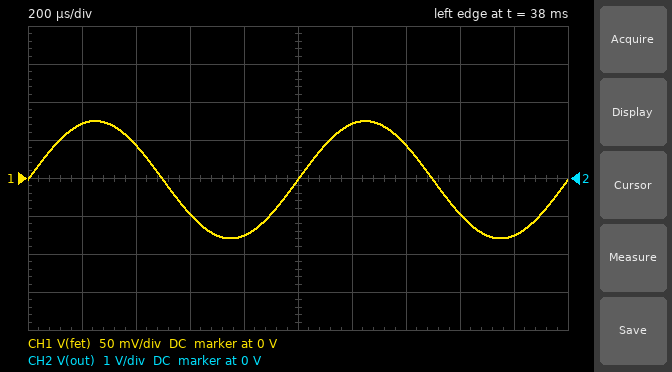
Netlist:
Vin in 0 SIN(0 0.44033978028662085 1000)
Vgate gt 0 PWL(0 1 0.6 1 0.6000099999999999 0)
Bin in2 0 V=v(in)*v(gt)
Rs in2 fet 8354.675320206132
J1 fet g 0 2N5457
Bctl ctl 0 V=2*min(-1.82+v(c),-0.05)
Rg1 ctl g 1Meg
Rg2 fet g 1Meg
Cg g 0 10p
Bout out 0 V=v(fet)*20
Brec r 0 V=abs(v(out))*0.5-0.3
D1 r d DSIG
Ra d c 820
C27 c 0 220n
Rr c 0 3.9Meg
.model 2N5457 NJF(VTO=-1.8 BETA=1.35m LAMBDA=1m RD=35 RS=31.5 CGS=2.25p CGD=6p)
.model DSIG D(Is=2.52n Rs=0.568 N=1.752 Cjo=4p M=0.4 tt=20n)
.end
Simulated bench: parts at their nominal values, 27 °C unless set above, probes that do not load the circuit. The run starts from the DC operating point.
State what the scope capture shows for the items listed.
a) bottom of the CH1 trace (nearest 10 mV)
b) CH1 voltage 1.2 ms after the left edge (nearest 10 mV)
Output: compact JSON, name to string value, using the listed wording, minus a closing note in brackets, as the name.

{"bottom of the CH1 trace": "-80 mV", "CH1 voltage 1.2 ms after the left edge": "70 mV"}
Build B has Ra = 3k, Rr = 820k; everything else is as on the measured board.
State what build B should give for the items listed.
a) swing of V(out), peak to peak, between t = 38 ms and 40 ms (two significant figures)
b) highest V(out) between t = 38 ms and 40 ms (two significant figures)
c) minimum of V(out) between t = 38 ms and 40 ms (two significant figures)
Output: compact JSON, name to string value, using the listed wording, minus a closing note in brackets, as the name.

{"swing of V(out), peak to peak, between t = 38 ms and 40 ms": "3.2 V", "highest V(out) between t = 38 ms and 40 ms": "1.6 V", "minimum of V(out) between t = 38 ms and 40 ms": "-1.7 V"}
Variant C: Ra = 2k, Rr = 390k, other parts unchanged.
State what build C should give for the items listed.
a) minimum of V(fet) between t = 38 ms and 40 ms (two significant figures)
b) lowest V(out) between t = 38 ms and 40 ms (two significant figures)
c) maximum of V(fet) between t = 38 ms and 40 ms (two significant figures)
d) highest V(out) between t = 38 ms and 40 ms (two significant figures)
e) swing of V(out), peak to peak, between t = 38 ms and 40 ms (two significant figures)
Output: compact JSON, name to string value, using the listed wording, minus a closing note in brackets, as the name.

{"minimum of V(fet) between t = 38 ms and 40 ms": "-86 mV", "lowest V(out) between t = 38 ms and 40 ms": "-1.7 V", "maximum of V(fet) between t = 38 ms and 40 ms": "81 mV", "highest V(out) between t = 38 ms and 40 ms": "1.6 V", "swing of V(out), peak to peak, between t = 38 ms and 40 ms": "3.3 V"}
